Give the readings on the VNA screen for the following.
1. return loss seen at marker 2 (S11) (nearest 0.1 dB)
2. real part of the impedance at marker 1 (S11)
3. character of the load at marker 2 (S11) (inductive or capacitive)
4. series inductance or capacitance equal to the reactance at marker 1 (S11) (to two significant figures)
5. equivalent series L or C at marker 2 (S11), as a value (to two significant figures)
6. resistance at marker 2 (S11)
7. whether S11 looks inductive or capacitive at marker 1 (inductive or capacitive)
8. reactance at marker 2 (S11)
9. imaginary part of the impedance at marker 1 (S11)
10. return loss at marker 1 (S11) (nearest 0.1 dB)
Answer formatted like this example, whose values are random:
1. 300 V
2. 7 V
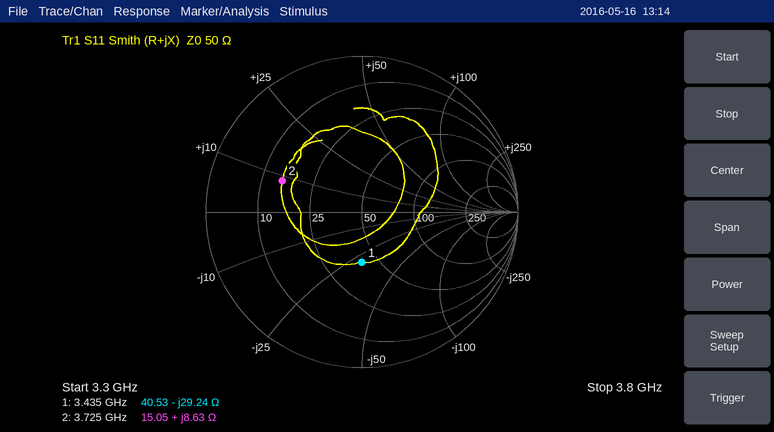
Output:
1. 5.2 dB
2. 40.53 Ω
3. inductive
4. 1.6 pF
5. 370 pH
6. 15.05 Ω
7. capacitive
8. +8.63 Ω
9. -29.24 Ω
10. 9.8 dB
